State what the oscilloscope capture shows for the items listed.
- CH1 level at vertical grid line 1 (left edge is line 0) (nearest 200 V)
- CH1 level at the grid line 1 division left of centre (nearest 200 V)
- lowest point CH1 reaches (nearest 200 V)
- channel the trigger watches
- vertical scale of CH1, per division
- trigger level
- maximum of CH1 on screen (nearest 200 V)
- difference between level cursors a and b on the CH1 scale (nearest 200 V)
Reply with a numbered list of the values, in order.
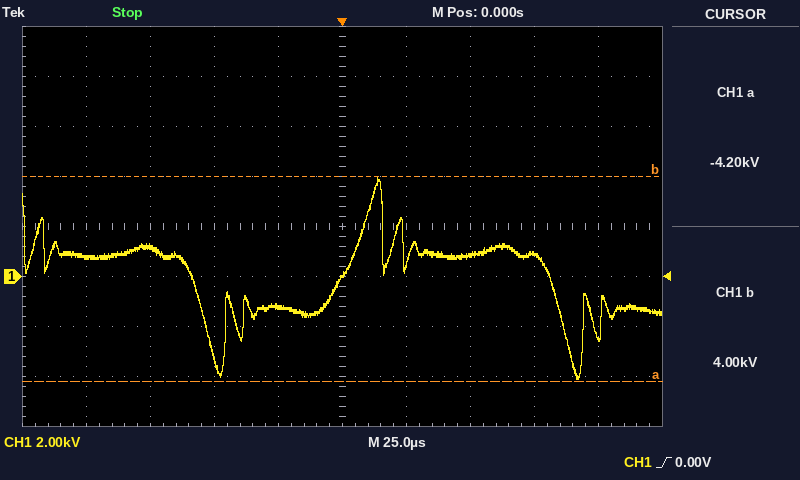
1. 800 V
2. -1.2 kV
3. -4.2 kV
4. CH1
5. 2 kV
6. 0.00 V
7. 4.0 kV
8. 8.2 kV
